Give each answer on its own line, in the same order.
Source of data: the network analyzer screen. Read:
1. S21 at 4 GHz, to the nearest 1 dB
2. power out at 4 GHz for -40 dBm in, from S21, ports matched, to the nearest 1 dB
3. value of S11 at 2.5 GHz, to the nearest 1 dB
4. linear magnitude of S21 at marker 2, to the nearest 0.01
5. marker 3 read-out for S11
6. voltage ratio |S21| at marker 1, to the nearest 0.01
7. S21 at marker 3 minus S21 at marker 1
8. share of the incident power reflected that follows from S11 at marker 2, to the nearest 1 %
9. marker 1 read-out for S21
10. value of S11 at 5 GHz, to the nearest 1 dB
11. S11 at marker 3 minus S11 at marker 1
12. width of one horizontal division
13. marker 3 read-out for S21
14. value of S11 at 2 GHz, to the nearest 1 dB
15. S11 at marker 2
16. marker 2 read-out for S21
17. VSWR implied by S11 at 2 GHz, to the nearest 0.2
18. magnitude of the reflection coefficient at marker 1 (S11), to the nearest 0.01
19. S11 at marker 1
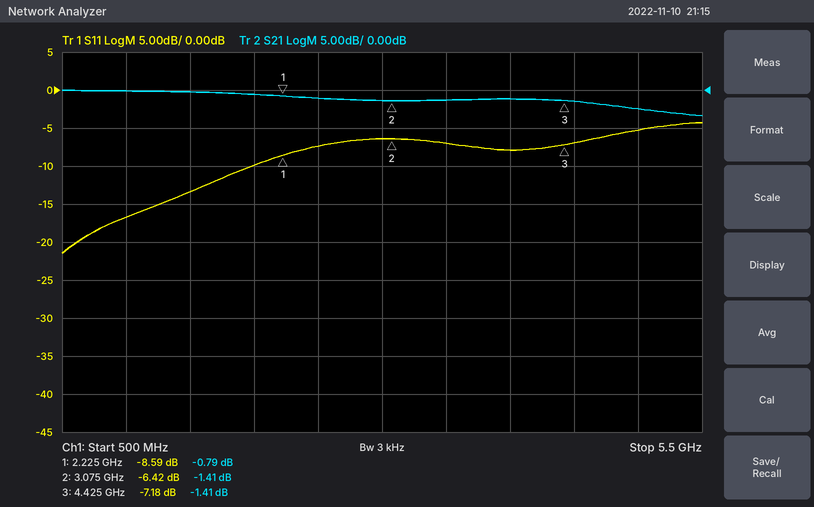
-1 dB
-41 dBm
-7 dB
0.85
-7.18 dB
0.91
-0.62 dB
23 %
-0.79 dB
-5 dB
1.41 dB
500 MHz
-1.41 dB
-10 dB
-6.42 dB
-1.41 dB
2.0
0.37
-8.59 dB
